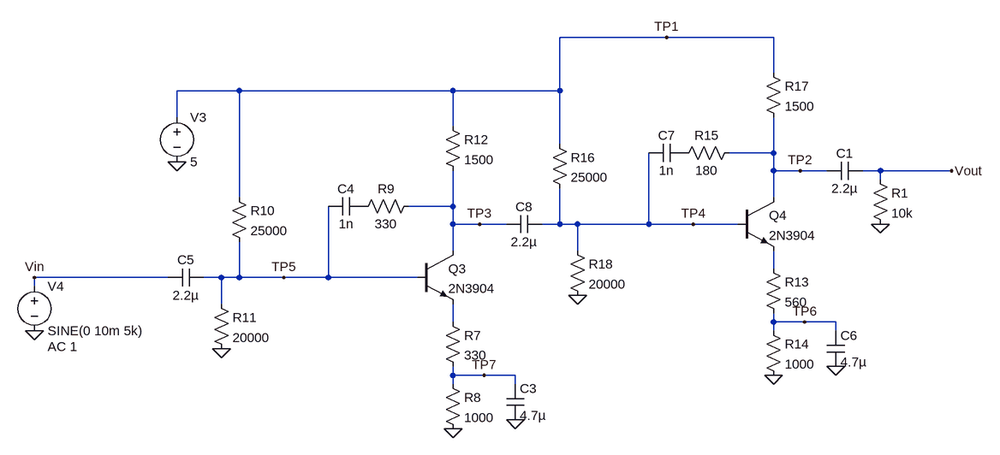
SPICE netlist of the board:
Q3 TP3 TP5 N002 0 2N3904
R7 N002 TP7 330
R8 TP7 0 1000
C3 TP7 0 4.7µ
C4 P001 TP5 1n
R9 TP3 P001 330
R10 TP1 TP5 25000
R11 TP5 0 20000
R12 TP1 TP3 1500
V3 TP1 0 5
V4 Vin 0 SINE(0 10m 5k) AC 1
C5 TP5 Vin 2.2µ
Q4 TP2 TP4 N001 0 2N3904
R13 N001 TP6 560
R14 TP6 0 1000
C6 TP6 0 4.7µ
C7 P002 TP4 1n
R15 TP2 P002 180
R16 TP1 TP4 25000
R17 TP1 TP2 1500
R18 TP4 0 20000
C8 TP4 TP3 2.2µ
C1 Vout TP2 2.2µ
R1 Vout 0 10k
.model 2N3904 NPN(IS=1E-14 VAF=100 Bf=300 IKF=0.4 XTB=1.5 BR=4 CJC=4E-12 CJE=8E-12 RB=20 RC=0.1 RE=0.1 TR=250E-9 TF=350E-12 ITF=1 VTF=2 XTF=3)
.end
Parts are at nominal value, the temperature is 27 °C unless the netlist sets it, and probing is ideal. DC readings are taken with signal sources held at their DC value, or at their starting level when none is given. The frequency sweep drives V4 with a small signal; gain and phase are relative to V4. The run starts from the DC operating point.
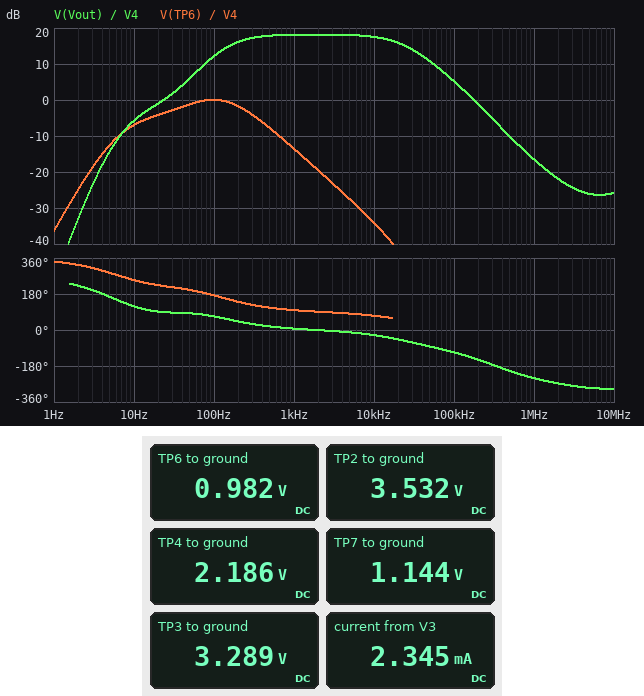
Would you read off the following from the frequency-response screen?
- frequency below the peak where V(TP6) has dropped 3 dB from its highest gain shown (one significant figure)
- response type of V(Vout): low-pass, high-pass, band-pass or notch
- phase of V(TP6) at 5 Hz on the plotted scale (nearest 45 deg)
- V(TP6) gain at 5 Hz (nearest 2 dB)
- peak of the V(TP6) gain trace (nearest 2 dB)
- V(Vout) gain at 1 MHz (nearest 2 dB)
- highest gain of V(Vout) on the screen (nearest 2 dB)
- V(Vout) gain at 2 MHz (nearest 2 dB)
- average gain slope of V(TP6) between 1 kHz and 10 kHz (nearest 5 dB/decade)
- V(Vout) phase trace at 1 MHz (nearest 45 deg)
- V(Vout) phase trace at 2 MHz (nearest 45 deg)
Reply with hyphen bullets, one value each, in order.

- 30 Hz
- band-pass
- 270 deg
- -12 dB
- 0 dB
- -16 dB
- 18 dB
- -22 dB
- -20 dB/decade
- -225 deg
- -270 deg
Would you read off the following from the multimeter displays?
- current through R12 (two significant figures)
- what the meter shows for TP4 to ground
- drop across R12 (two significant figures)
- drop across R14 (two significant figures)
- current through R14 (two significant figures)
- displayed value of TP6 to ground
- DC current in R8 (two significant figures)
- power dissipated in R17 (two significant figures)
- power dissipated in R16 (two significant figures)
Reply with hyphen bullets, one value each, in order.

- 1.1 mA
- 2.186 V
- 1.7 V
- 980 mV
- 980 µA
- 0.982 V
- 1.1 mA
- 1.4 mW
- 320 µW
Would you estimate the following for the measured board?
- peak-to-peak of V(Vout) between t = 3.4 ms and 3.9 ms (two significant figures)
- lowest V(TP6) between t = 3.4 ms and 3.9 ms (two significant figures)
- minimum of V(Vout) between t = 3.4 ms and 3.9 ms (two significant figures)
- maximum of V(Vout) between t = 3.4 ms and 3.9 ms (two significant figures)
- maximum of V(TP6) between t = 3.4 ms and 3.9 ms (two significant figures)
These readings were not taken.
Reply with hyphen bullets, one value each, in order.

- 160 mV
- 980 mV
- -80 mV
- 80 mV
- 980 mV
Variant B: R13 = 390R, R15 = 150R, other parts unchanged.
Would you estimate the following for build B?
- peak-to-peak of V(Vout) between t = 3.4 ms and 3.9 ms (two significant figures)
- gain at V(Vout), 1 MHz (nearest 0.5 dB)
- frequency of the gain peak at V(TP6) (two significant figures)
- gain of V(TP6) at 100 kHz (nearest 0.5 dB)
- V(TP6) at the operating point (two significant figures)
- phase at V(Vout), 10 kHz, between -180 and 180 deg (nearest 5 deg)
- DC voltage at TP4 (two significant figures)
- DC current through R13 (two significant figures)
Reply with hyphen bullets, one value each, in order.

- 220 mV
- -17.5 dB
- 110 Hz
- -62.5 dB
- 1.1 V
- -30 deg
- 2.2 V
- 1.1 mA
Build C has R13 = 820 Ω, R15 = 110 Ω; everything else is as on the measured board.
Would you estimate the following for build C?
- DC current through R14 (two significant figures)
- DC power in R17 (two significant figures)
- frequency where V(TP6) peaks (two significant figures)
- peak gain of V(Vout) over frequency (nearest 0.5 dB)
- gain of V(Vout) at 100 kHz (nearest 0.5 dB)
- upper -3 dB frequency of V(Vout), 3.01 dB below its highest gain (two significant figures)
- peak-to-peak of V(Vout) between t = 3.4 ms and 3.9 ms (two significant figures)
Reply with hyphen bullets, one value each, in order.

- 850 µA
- 1.1 mW
- 85 Hz
- 15.0 dB
- 4.0 dB
- 28 kHz
- 110 mV
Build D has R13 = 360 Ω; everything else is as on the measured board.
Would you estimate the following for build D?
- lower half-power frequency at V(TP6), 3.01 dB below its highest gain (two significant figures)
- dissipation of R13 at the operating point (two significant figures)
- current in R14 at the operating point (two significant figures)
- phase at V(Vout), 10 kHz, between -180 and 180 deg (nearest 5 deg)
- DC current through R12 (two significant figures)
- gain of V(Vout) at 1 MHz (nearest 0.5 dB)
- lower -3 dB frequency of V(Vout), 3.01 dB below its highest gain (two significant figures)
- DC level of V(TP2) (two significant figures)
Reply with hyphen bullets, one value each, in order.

- 39 Hz
- 450 µW
- 1.1 mA
- -30 deg
- 1.1 mA
- -18.5 dB
- 180 Hz
- 3.3 V
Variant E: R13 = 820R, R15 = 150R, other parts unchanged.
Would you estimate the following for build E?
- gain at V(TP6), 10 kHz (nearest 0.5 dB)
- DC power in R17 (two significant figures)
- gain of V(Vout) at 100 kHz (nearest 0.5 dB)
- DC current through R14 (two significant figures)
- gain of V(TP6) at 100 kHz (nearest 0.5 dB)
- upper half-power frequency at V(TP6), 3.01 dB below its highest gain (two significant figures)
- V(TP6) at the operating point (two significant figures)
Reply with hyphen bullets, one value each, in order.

- -37.0 dB
- 1.1 mW
- 3.5 dB
- 850 µA
- -66.0 dB
- 230 Hz
- 850 mV
